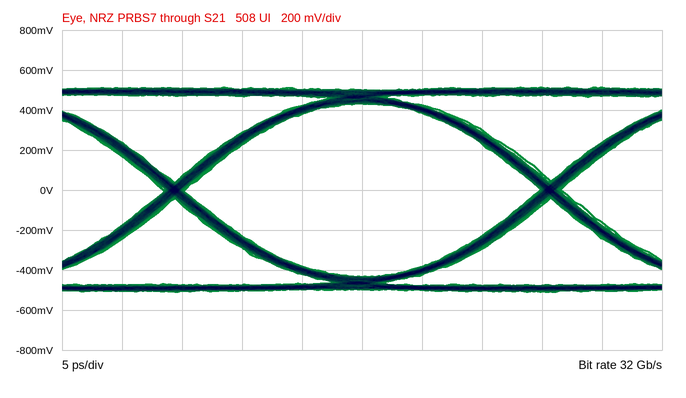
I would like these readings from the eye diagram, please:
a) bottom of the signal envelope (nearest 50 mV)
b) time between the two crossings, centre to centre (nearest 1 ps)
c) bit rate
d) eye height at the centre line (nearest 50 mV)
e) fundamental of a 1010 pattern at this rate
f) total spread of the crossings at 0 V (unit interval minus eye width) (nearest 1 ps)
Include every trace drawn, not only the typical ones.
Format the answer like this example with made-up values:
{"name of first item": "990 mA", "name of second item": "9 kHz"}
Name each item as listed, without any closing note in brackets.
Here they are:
{"bottom of the signal envelope": "-500 mV", "time between the two crossings, centre to centre": "31 ps", "bit rate": "32 Gb/s", "eye height at the centre line": "850 mV", "fundamental of a 1010 pattern at this rate": "16 GHz", "total spread of the crossings at 0 V (unit interval minus eye width)": "2 ps"}
